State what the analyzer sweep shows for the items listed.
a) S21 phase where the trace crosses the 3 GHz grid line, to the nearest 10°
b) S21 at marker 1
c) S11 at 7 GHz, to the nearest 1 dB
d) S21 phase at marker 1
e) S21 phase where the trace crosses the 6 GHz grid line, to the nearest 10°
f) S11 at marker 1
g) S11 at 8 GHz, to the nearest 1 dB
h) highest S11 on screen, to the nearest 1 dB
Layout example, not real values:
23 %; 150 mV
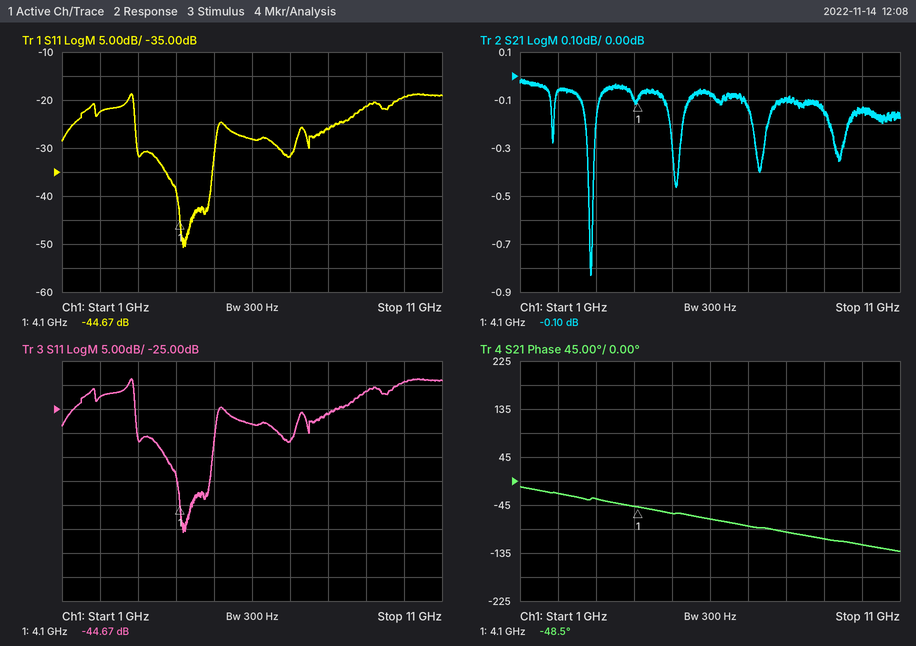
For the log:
-30°; -0.10 dB; -32 dB; -48.5°; -70°; -44.67 dB; -26 dB; -19 dB
